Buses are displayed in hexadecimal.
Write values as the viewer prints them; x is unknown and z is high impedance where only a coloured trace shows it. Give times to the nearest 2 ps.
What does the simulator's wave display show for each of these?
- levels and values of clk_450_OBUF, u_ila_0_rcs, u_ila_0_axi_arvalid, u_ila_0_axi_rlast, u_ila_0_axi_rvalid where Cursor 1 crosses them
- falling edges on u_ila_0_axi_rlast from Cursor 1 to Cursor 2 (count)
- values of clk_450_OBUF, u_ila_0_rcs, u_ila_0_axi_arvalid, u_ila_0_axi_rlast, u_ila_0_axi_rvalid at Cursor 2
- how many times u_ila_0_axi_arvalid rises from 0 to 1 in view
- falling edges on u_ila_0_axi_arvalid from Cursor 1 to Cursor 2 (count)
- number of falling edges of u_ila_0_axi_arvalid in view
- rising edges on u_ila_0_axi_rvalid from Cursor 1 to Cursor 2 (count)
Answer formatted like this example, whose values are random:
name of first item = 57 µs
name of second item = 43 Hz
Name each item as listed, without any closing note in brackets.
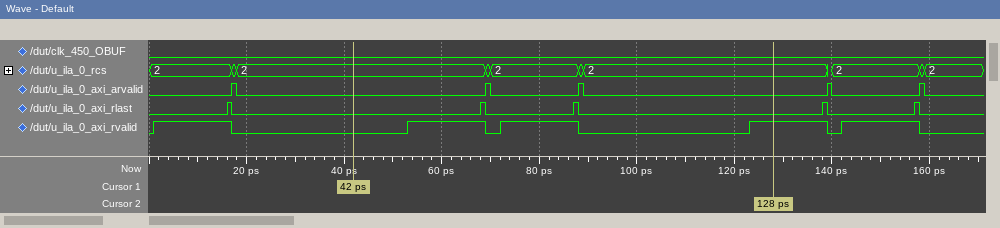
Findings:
levels and values of clk_450_OBUF, u_ila_0_rcs, u_ila_0_axi_arvalid, u_ila_0_axi_rlast, u_ila_0_axi_rvalid where Cursor 1 crosses them = clk_450_OBUF=0, u_ila_0_rcs=2, u_ila_0_axi_arvalid=0, u_ila_0_axi_rlast=0, u_ila_0_axi_rvalid=0
falling edges on u_ila_0_axi_rlast from Cursor 1 to Cursor 2 = 2
values of clk_450_OBUF, u_ila_0_rcs, u_ila_0_axi_arvalid, u_ila_0_axi_rlast, u_ila_0_axi_rvalid at Cursor 2 = clk_450_OBUF=0, u_ila_0_rcs=2, u_ila_0_axi_arvalid=0, u_ila_0_axi_rlast=0, u_ila_0_axi_rvalid=1
how many times u_ila_0_axi_arvalid rises from 0 to 1 in view = 5
falling edges on u_ila_0_axi_arvalid from Cursor 1 to Cursor 2 = 2
number of falling edges of u_ila_0_axi_arvalid in view = 5
rising edges on u_ila_0_axi_rvalid from Cursor 1 to Cursor 2 = 3
